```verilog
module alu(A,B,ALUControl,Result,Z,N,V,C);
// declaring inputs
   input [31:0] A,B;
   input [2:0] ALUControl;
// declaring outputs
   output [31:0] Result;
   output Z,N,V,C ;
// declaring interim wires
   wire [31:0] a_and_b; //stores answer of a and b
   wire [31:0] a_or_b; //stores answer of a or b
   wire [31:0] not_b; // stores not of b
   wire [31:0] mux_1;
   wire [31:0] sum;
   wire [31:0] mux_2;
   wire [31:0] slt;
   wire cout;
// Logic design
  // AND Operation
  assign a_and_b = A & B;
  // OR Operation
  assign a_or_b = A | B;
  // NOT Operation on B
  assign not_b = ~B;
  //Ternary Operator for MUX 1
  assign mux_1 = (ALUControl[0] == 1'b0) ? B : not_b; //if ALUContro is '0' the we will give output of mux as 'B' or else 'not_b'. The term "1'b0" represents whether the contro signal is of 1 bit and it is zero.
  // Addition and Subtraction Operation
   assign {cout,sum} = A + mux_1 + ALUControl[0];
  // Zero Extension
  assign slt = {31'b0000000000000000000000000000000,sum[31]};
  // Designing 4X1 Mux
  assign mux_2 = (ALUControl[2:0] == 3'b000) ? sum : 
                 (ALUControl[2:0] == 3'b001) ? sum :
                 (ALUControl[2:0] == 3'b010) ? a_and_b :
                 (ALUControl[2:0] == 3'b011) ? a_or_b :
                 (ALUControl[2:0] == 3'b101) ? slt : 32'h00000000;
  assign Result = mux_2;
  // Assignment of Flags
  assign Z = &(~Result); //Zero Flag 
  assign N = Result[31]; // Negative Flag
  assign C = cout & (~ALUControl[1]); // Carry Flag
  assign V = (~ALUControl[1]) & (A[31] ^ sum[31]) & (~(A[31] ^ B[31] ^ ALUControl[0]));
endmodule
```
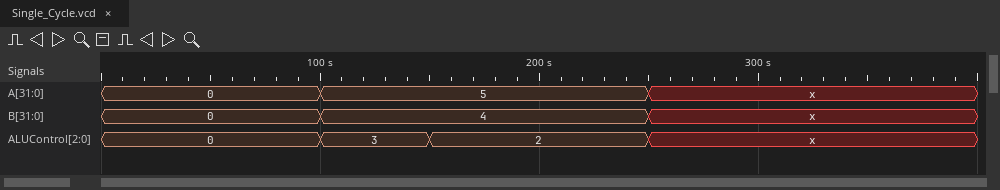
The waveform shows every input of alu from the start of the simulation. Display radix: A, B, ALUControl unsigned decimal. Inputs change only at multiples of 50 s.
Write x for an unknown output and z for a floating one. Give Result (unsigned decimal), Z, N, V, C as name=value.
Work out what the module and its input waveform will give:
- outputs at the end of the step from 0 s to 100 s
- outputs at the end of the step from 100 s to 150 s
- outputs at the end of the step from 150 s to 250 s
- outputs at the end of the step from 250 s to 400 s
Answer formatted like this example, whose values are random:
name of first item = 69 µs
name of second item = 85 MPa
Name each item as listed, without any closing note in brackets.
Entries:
outputs at the end of the step from 0 s to 100 s = Result=0, Z=1, N=0, V=0, C=0
outputs at the end of the step from 100 s to 150 s = Result=5, Z=0, N=0, V=0, C=0
outputs at the end of the step from 150 s to 250 s = Result=4, Z=0, N=0, V=0, C=0
outputs at the end of the step from 250 s to 400 s = Result=x, Z=x, N=x, V=x, C=x
